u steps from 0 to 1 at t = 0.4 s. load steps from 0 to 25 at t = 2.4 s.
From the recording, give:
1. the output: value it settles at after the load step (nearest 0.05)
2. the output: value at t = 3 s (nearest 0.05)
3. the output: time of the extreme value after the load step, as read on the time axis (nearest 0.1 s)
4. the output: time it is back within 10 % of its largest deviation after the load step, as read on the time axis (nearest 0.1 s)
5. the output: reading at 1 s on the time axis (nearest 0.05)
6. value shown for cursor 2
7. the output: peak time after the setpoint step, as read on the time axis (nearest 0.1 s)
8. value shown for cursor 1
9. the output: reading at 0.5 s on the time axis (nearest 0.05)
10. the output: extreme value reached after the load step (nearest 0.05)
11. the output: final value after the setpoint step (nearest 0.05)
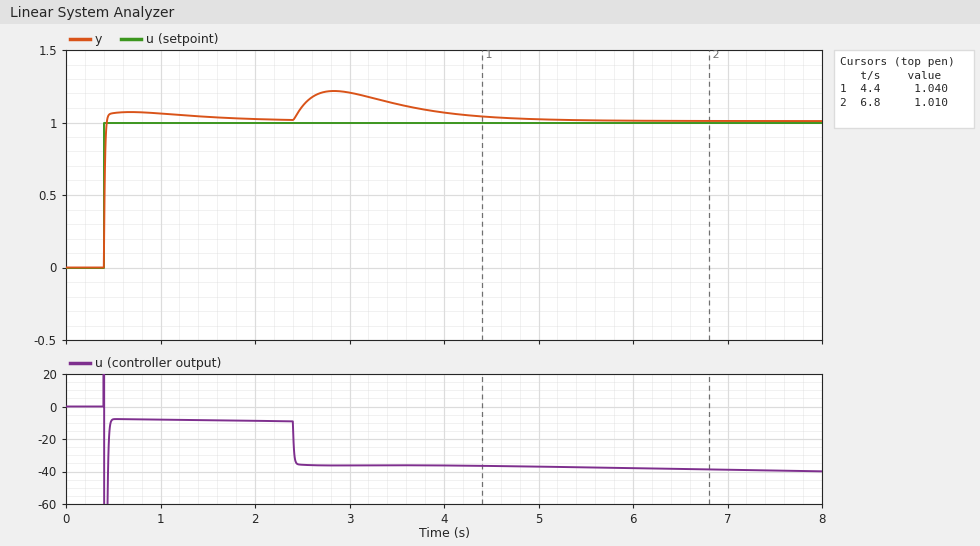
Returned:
1.00
1.20
2.8 s
4.7 s
1.05
1.010
0.7 s
1.040
1.05
1.20
1.00
